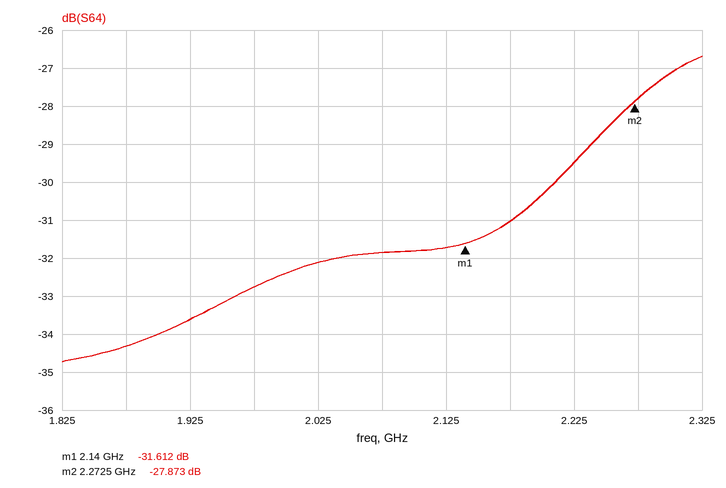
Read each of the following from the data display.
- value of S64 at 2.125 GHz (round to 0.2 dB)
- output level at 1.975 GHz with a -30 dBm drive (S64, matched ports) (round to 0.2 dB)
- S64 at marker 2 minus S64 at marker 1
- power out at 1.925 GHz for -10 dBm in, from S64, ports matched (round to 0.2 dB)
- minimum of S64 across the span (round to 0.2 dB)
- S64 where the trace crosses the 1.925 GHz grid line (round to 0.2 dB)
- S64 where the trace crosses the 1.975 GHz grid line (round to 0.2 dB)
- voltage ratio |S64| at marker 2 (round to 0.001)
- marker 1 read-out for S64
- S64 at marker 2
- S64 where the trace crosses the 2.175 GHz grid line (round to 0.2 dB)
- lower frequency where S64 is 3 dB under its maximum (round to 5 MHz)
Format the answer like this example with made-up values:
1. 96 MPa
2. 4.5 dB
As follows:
1. -31.8 dB
2. -62.8 dBm
3. 3.739 dB
4. -43.6 dBm
5. -34.8 dB
6. -33.6 dB
7. -32.8 dB
8. 0.040
9. -31.612 dB
10. -27.873 dB
11. -31.0 dB
12. 2.220 GHz
